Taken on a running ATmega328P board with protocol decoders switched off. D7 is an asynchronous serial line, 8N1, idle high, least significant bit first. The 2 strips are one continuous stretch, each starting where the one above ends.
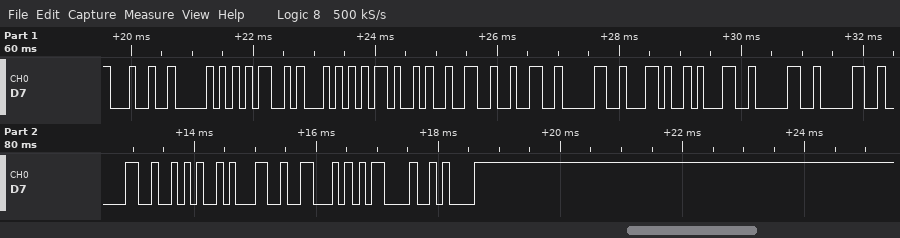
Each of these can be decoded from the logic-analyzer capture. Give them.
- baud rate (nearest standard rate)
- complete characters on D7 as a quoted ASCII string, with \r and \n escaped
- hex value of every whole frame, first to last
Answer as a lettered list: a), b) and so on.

a) 9600 baud
b) "$PMTK220,1000*1F\r\n"
c) 24 50 4D 54 4B 32 32 30 2C 31 30 30 30 2A 31 46 0D 0A
